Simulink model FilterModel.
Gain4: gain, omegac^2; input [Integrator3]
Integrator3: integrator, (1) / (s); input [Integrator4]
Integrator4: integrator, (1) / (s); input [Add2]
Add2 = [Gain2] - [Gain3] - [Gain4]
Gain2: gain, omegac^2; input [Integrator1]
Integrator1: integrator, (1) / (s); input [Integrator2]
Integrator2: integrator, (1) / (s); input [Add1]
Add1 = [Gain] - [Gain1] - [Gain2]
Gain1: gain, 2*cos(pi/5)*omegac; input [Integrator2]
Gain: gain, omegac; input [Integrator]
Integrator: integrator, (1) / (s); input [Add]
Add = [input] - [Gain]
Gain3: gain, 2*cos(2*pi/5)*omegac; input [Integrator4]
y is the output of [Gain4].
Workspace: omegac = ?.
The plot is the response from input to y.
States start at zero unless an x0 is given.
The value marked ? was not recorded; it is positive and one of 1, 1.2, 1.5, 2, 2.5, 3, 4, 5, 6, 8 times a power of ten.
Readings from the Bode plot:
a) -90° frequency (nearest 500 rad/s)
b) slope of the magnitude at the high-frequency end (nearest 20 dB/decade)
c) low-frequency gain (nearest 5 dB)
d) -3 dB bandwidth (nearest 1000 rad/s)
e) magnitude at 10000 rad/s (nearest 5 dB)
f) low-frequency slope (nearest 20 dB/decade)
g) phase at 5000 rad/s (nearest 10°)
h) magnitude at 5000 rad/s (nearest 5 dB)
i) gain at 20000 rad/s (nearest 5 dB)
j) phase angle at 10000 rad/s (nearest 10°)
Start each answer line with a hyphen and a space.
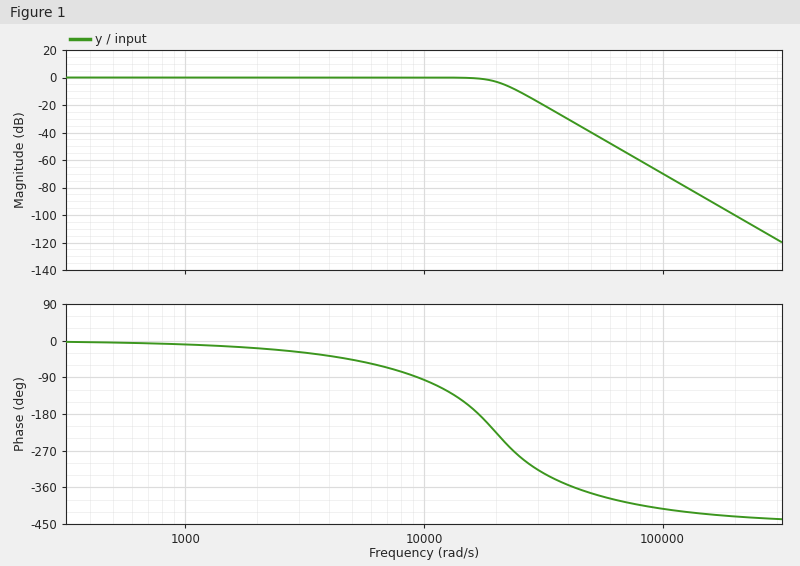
- 9500 rad/s
- -100 dB/decade
- 0 dB
- 20000 rad/s
- 0 dB
- 0 dB/decade
- -50°
- 0 dB
- -5 dB
- -100°
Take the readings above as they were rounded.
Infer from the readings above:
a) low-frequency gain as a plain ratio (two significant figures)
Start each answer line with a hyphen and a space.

- 1.0
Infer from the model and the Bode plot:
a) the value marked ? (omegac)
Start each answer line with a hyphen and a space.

- 20000
